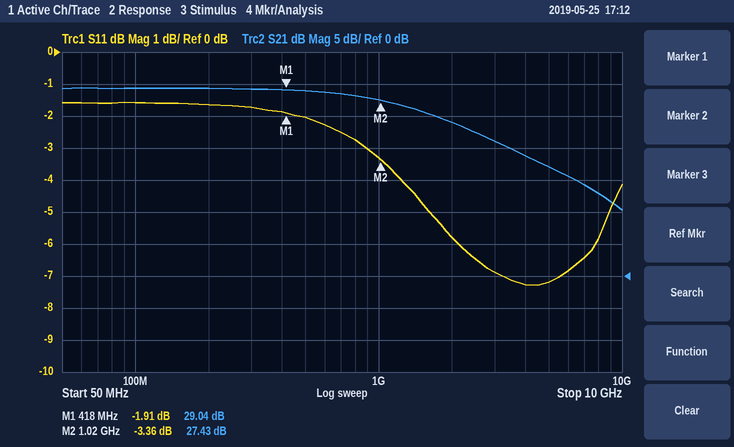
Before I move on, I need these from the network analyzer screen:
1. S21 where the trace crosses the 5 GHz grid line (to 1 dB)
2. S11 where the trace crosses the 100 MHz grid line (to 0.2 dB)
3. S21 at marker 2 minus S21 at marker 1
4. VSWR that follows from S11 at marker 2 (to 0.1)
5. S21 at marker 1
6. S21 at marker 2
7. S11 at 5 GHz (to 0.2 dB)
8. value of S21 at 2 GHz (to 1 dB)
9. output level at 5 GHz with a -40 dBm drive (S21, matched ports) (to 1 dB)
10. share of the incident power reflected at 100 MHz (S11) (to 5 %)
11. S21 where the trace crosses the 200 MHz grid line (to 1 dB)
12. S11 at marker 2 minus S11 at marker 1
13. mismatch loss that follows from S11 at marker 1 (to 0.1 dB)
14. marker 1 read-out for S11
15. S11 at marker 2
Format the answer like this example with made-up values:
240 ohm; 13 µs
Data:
17 dB; -1.6 dB; -1.61 dB; 5.2; 29.04 dB; 27.43 dB; -7.2 dB; 24 dB; -23 dBm; 70 %; 29 dB; -1.45 dB; 4.5 dB; -1.91 dB; -3.36 dB
